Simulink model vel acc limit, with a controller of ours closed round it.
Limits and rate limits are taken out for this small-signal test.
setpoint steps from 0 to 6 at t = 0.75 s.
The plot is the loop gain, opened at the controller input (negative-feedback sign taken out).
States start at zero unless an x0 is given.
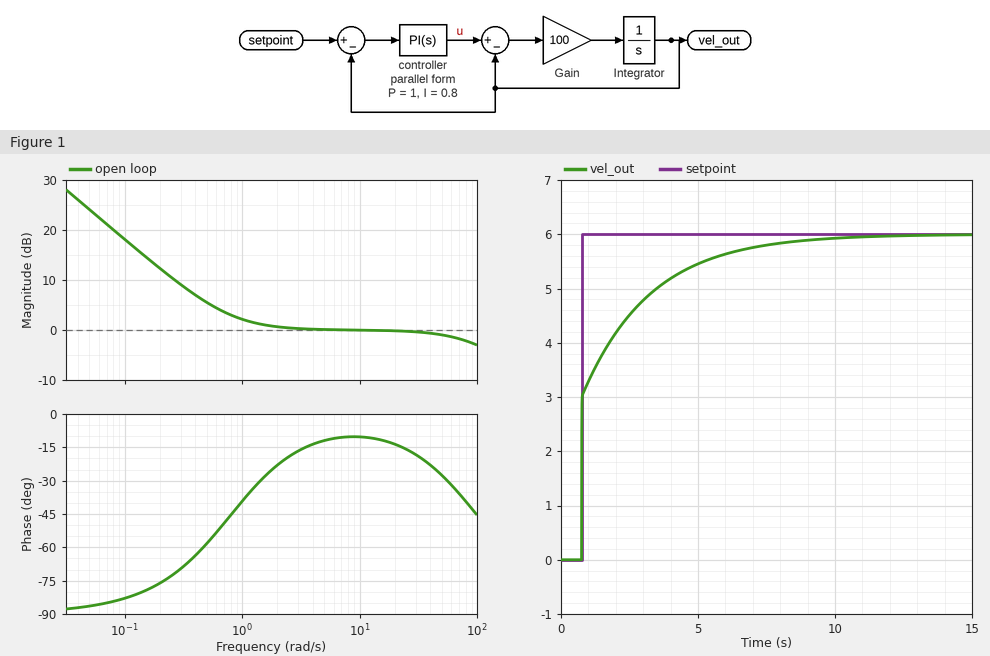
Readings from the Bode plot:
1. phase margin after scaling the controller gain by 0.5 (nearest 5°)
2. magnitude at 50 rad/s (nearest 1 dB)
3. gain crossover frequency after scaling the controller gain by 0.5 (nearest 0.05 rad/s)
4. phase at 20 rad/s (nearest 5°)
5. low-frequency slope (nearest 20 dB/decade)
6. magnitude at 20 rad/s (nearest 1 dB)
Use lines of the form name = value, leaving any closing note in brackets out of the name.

phase margin after scaling the controller gain by 0.5 = 120°
magnitude at 50 rad/s = -1 dB
gain crossover frequency after scaling the controller gain by 0.5 = 0.45 rad/s
phase at 20 rad/s = -15°
low-frequency slope = -20 dB/decade
magnitude at 20 rad/s = 0 dB
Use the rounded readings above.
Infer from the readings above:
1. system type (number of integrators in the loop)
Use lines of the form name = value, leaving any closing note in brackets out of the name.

system type = 1
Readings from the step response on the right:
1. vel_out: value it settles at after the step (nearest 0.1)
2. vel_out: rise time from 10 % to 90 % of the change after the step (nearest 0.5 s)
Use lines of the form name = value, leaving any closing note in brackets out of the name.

vel_out: value it settles at after the step = 6.0
vel_out: rise time from 10 % to 90 % of the change after the step = 4.0 s
